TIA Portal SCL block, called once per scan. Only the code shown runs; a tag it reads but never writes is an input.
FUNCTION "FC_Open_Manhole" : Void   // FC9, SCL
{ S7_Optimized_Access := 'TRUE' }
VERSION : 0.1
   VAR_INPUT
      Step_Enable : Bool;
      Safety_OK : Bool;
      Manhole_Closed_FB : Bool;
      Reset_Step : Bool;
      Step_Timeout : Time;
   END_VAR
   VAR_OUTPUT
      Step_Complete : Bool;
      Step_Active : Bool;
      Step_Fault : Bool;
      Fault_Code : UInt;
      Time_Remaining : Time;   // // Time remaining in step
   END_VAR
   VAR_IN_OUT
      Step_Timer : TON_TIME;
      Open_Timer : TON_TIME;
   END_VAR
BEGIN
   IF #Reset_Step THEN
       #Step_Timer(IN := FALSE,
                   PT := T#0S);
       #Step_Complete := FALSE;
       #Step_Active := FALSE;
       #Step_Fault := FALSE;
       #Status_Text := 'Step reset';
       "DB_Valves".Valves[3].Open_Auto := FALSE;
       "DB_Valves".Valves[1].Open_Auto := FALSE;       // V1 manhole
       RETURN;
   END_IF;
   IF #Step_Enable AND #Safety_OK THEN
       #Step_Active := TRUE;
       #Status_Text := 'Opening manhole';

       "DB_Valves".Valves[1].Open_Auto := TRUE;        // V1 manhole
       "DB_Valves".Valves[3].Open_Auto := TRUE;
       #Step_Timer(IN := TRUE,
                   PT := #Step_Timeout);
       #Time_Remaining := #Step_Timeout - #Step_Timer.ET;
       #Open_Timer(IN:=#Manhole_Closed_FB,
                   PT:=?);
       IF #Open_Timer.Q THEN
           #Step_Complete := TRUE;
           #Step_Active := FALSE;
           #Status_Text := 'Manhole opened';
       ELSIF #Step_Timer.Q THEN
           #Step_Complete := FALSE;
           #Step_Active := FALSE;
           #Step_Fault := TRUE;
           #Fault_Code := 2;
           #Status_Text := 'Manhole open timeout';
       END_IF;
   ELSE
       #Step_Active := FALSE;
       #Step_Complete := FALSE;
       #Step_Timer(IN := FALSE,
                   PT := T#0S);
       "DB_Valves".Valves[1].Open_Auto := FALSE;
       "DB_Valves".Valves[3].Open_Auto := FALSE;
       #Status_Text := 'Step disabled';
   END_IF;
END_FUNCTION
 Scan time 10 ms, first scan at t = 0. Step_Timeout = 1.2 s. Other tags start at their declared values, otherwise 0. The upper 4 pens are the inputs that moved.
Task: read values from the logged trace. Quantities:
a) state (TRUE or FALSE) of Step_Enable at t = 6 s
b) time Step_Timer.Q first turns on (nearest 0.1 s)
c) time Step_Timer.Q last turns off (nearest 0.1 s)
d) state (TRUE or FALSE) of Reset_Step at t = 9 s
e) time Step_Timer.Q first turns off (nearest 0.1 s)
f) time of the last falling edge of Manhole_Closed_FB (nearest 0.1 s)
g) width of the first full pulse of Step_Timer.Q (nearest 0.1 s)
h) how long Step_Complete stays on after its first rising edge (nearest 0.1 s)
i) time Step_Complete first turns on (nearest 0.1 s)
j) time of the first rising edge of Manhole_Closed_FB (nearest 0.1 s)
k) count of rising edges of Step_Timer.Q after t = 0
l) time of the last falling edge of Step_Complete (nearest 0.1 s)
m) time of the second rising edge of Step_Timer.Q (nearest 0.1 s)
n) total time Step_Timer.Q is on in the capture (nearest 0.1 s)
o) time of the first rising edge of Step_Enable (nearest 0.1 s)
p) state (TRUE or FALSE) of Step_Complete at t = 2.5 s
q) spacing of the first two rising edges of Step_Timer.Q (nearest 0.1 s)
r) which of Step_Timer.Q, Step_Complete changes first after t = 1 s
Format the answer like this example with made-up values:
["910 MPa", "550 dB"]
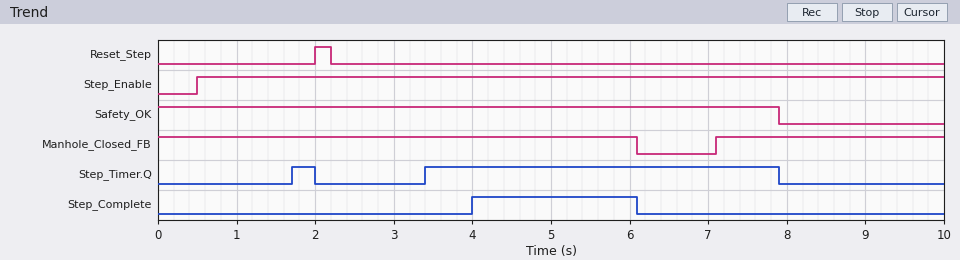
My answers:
["TRUE", "1.7 s", "7.9 s", "FALSE", "2.0 s", "6.1 s", "0.3 s", "2.1 s", "4.0 s", "7.1 s", "2", "6.1 s", "3.4 s", "4.8 s", "0.5 s", "FALSE", "1.7 s", "Step_Timer.Q"]
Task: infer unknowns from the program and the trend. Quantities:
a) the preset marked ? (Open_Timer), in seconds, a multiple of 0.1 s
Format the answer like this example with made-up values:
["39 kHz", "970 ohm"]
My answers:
["3.5 s"]
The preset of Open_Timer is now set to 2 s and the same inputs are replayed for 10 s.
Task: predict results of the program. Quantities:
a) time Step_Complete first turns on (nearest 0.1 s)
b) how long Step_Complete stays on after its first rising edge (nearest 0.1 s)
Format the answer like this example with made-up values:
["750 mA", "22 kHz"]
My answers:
["2.5 s", "3.6 s"]
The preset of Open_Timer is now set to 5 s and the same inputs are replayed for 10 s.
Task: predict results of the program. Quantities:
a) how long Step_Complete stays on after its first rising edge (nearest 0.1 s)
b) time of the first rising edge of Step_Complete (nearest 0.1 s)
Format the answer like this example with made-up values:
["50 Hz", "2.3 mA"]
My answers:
["0.6 s", "5.5 s"]
